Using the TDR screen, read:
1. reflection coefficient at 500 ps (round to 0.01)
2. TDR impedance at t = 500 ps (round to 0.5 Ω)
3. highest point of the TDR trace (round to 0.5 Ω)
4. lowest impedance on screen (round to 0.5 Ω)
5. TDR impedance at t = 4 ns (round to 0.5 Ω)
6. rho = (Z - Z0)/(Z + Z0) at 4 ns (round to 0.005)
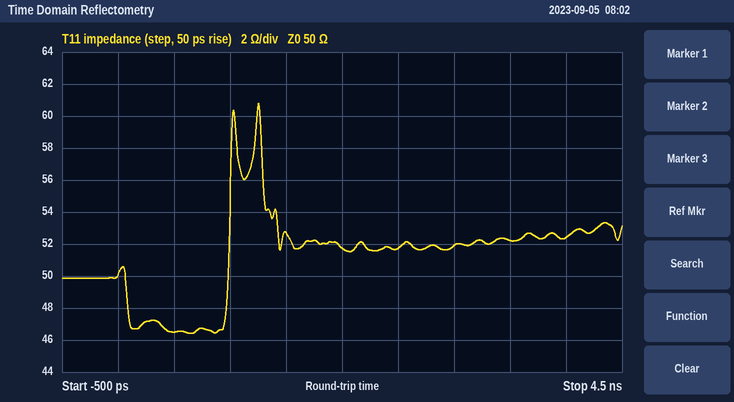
-0.04
46.5 Ω
61.0 Ω
46.5 Ω
52.5 Ω
+0.025
